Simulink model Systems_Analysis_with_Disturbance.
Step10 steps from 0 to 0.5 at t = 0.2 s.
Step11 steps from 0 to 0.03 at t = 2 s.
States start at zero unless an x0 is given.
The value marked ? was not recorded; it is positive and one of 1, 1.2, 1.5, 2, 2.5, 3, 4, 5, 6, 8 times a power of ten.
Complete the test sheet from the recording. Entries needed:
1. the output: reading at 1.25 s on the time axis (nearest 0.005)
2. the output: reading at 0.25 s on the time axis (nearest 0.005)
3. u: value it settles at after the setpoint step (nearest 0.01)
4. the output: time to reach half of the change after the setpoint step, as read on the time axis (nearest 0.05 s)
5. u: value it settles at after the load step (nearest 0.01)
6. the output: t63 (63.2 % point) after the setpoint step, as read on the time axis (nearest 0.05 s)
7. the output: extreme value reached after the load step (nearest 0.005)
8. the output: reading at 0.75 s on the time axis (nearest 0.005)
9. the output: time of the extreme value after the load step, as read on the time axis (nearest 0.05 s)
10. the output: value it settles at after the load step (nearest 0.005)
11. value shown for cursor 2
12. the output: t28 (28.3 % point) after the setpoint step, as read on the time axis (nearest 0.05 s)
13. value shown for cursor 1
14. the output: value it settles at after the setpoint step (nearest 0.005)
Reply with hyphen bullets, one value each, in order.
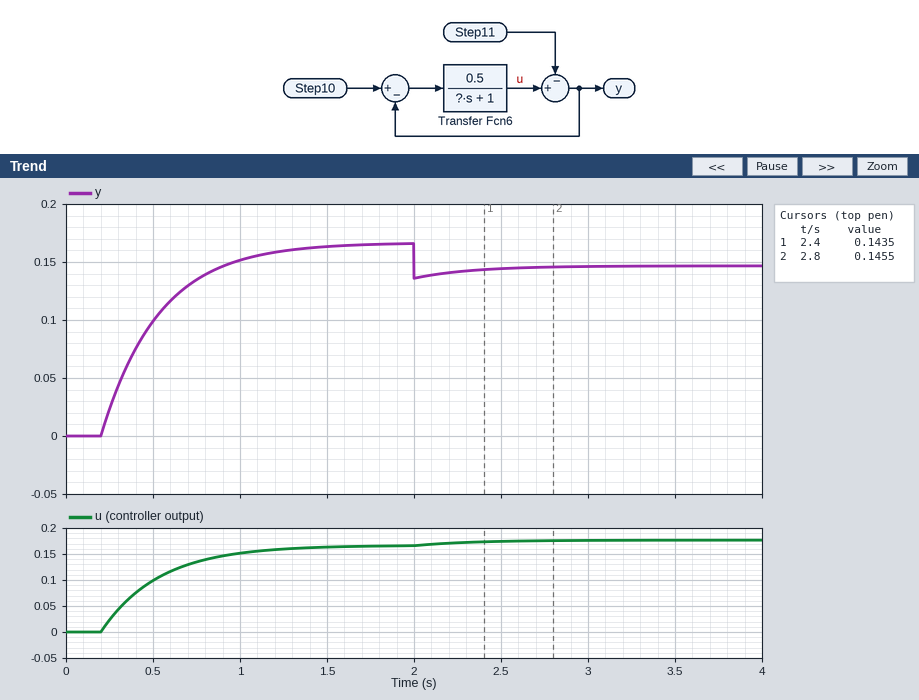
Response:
- 0.160
- 0.025
- 0.17
- 0.45 s
- 0.18
- 0.55 s
- 0.135
- 0.135
- 2.00 s
- 0.145
- 0.1455
- 0.30 s
- 0.1435
- 0.165
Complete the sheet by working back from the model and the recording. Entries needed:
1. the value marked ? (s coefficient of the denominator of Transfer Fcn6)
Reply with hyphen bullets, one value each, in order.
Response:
- 0.5
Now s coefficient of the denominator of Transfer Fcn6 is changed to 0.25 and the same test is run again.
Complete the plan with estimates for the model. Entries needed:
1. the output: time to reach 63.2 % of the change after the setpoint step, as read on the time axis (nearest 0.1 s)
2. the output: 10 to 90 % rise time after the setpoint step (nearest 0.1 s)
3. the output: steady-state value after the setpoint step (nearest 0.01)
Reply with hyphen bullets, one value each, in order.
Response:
- 0.4 s
- 0.4 s
- 0.17
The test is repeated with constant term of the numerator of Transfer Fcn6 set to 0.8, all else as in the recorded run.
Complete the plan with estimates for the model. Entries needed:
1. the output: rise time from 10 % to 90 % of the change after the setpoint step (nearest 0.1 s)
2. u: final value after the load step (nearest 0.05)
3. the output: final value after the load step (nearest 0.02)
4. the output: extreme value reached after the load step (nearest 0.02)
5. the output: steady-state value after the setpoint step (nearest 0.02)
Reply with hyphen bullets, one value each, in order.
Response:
- 0.6 s
- 0.25
- 0.20
- 0.20
- 0.22
